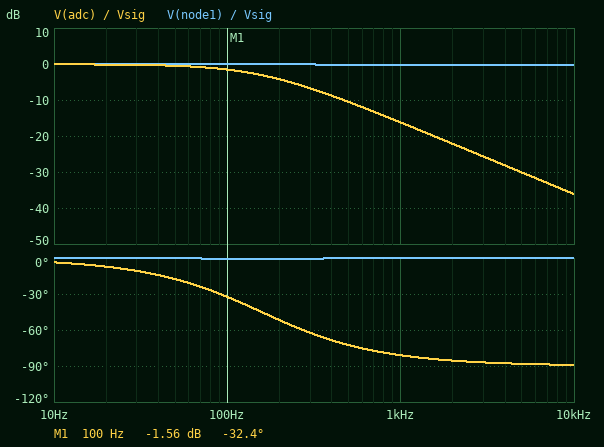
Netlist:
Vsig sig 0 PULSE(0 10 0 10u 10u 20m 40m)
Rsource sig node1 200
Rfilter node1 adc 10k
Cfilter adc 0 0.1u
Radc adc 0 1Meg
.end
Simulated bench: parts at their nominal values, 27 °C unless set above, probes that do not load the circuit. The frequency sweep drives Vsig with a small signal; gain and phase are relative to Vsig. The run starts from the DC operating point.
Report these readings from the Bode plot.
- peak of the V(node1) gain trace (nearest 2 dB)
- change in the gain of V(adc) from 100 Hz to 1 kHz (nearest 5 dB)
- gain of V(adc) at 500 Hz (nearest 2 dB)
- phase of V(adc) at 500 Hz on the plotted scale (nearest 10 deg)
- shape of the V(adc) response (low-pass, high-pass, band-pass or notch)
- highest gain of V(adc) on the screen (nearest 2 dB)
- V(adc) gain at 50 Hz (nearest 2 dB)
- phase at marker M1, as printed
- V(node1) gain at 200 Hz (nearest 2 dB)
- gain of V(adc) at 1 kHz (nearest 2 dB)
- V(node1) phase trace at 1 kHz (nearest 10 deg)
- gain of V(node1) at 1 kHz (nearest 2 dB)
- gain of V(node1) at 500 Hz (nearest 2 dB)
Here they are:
0 dB
-15 dB
-10 dB
-70 deg
low-pass
0 dB
0 dB
-32.4 deg
0 dB
-16 dB
0 deg
0 dB
0 dB
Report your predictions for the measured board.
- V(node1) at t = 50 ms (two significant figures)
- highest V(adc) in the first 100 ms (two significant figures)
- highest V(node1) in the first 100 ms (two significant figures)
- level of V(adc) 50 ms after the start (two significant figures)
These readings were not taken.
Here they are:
10 V
9.9 V
10 V
9.9 V
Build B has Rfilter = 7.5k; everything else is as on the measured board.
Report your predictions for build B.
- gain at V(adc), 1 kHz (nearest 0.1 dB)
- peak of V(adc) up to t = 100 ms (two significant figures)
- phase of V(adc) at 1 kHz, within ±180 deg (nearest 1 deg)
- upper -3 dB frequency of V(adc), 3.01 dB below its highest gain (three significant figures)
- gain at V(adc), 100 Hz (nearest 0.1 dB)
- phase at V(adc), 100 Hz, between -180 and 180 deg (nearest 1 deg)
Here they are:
-13.9 dB
9.9 V
-78 deg
208 Hz
-1.0 dB
-26 deg
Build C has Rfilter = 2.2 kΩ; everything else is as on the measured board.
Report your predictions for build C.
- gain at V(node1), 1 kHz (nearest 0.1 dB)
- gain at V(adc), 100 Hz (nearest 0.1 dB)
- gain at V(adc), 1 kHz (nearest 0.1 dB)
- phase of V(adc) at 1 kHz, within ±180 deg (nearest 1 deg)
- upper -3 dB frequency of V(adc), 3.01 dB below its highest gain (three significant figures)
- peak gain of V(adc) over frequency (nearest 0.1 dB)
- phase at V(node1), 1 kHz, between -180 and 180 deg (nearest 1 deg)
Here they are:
-0.5 dB
-0.1 dB
-5.2 dB
-56 deg
665 Hz
0 dB
-2 deg
